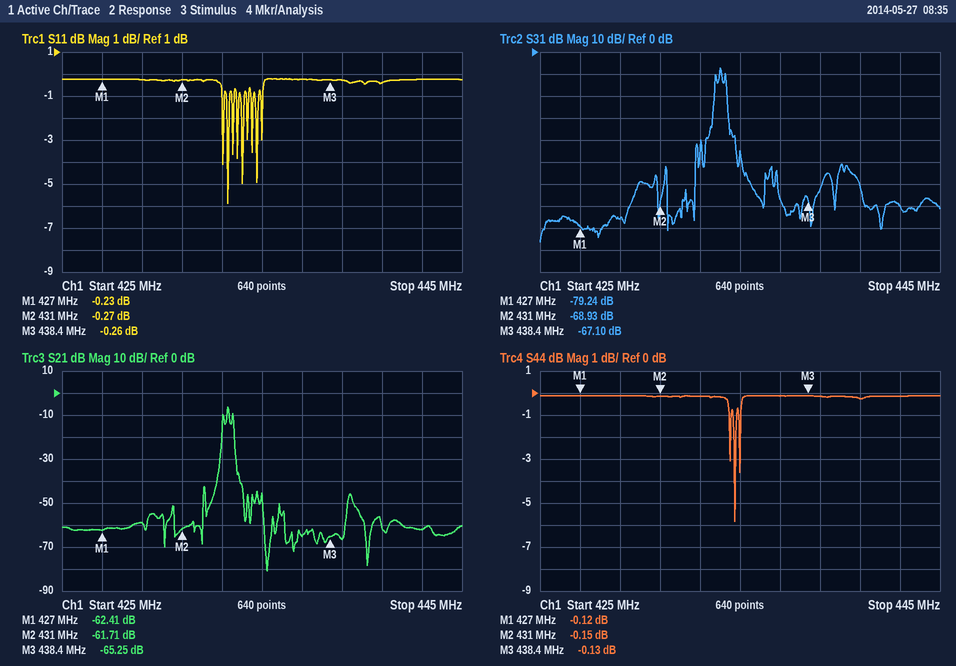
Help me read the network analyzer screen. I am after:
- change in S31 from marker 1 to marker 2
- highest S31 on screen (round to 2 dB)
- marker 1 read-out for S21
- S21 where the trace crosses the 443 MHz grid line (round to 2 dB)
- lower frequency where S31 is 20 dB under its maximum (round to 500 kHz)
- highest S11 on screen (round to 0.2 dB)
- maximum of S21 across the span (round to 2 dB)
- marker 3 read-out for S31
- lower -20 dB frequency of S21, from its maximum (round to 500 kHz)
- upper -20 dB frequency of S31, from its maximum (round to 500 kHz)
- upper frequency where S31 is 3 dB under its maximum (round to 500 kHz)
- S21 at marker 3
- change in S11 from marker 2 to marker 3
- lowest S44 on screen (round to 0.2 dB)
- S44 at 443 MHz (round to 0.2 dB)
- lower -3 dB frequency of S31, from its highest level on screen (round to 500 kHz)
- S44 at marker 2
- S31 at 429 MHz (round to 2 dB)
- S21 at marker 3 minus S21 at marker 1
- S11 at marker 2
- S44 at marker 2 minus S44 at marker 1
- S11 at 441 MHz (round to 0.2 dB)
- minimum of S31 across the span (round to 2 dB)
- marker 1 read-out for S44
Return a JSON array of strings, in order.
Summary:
["10.31 dB", "-8 dB", "-62.41 dB", "-62 dB", "433.5 MHz", "-0.2 dB", "-6 dB", "-67.10 dB", "433.0 MHz", "434.5 MHz", "434.0 MHz", "-65.25 dB", "0.01 dB", "-5.8 dB", "-0.2 dB", "434.0 MHz", "-0.15 dB", "-76 dB", "-2.84 dB", "-0.27 dB", "-0.03 dB", "-0.4 dB", "-86 dB", "-0.12 dB"]
